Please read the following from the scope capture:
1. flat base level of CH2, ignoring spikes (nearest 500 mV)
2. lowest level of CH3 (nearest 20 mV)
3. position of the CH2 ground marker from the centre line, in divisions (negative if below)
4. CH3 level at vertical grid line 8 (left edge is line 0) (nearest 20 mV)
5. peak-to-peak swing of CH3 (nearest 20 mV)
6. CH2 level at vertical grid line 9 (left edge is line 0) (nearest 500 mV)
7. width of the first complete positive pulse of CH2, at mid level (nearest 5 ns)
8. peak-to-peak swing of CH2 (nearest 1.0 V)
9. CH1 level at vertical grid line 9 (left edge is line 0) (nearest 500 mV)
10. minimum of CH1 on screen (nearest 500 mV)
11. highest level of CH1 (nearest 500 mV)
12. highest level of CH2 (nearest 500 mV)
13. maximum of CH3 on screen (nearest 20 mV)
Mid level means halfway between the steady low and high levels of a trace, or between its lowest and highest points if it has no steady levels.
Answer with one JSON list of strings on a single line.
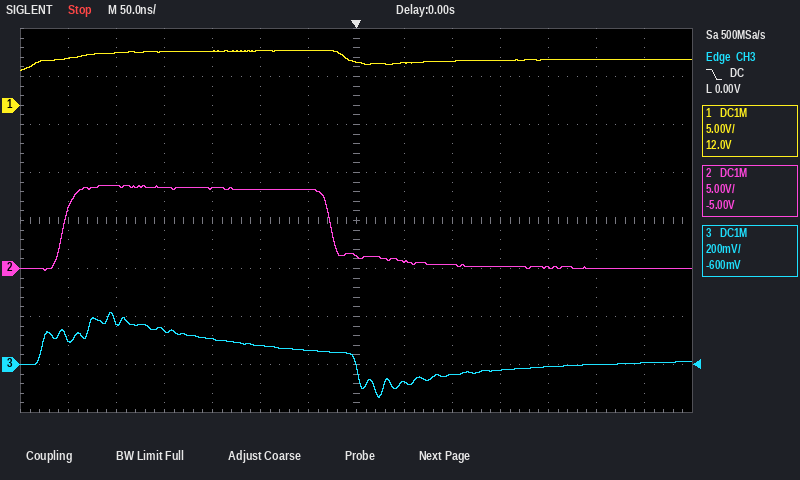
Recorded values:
["0.0 V", "-140 mV", "-1.0 div", "-80 mV", "360 mV", "500 mV", "280 ns", "9.0 V", "4.5 V", "3.5 V", "5.5 V", "8.5 V", "220 mV"]
